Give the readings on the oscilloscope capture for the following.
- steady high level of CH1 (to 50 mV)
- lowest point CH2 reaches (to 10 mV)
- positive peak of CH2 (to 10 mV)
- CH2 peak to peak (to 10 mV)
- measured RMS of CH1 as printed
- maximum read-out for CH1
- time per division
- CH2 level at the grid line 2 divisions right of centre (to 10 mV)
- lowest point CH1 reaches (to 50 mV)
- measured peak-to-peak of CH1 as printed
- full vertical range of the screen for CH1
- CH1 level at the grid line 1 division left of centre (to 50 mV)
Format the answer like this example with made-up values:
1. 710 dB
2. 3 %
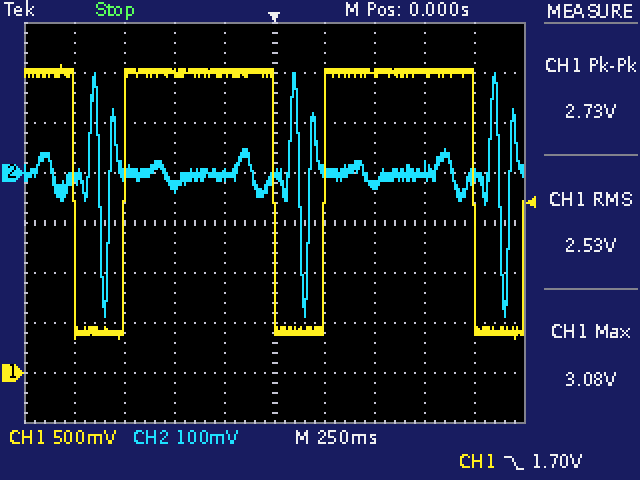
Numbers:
1. 3.00 V
2. -290 mV
3. 200 mV
4. 490 mV
5. 2.53 V
6. 3.08 V
7. 250 ms
8. -20 mV
9. 350 mV
10. 2.73 V
11. 4 V
12. 3.00 V
